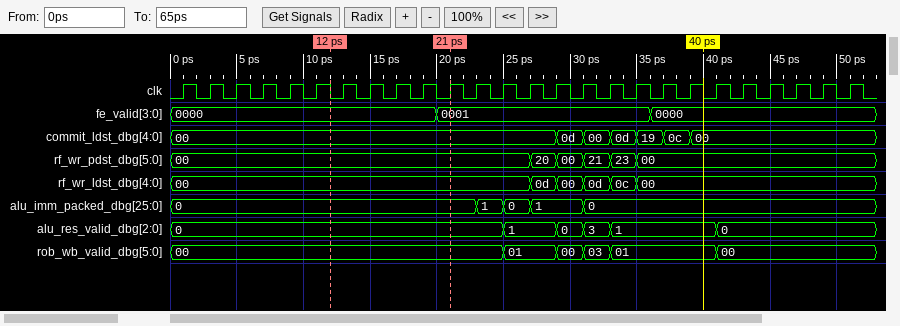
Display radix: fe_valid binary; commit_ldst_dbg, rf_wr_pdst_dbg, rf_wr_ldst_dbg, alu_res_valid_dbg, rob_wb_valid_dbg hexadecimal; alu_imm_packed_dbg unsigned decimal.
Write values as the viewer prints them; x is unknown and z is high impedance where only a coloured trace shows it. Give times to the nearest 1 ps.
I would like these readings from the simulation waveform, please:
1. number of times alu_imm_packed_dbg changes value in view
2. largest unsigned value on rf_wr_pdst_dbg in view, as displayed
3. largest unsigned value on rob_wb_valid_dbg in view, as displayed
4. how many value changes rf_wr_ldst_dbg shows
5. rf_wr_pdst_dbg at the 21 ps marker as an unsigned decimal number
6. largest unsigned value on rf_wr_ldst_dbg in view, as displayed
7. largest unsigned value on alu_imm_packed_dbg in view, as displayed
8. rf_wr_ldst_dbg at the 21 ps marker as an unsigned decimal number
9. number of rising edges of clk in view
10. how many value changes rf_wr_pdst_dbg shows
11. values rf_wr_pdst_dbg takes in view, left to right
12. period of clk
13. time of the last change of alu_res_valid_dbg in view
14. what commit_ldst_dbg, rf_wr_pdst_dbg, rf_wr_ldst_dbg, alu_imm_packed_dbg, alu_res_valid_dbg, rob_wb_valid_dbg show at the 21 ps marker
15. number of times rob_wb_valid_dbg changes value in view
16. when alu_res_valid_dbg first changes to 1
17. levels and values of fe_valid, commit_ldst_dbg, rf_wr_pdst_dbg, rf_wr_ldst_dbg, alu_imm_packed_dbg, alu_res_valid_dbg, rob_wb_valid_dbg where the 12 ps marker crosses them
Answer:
4
23
03
5
0
0d
1
0
26
5
00, 20, 00, 21, 23, 00
2 ps
41 ps
commit_ldst_dbg=00, rf_wr_pdst_dbg=00, rf_wr_ldst_dbg=00, alu_imm_packed_dbg=0, alu_res_valid_dbg=0, rob_wb_valid_dbg=00
5
25 ps
fe_valid=0000, commit_ldst_dbg=00, rf_wr_pdst_dbg=00, rf_wr_ldst_dbg=00, alu_imm_packed_dbg=0, alu_res_valid_dbg=0, rob_wb_valid_dbg=00
